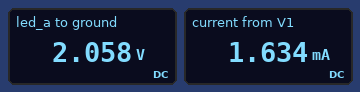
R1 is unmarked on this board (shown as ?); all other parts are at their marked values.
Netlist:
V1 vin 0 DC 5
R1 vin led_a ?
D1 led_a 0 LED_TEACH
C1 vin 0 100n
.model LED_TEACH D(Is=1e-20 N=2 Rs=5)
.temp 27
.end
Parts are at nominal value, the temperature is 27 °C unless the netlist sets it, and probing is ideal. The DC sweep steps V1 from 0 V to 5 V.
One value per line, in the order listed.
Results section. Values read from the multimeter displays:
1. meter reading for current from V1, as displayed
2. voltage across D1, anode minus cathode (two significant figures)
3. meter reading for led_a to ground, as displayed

1.634 mA
2.1 V
2.058 V
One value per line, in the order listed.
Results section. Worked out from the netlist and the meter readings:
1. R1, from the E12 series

1.8 kΩ
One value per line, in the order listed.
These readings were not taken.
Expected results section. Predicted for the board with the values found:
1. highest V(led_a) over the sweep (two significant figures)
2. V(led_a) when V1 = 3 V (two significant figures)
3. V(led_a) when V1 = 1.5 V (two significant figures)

2.1 V
2.0 V
1.5 V
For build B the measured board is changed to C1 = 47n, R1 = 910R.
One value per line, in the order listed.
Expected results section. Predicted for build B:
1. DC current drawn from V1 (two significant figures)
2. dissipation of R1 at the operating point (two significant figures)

3.2 mA
9.2 mW
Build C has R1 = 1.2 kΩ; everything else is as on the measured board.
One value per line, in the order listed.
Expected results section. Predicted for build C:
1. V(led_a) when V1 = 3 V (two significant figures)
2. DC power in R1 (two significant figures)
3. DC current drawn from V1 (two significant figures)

2.0 V
7.1 mW
2.4 mA
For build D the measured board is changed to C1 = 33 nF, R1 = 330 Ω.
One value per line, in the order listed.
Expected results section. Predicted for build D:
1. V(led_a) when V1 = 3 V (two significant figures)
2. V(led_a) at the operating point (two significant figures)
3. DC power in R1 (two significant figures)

2.1 V
2.2 V
24 mW
